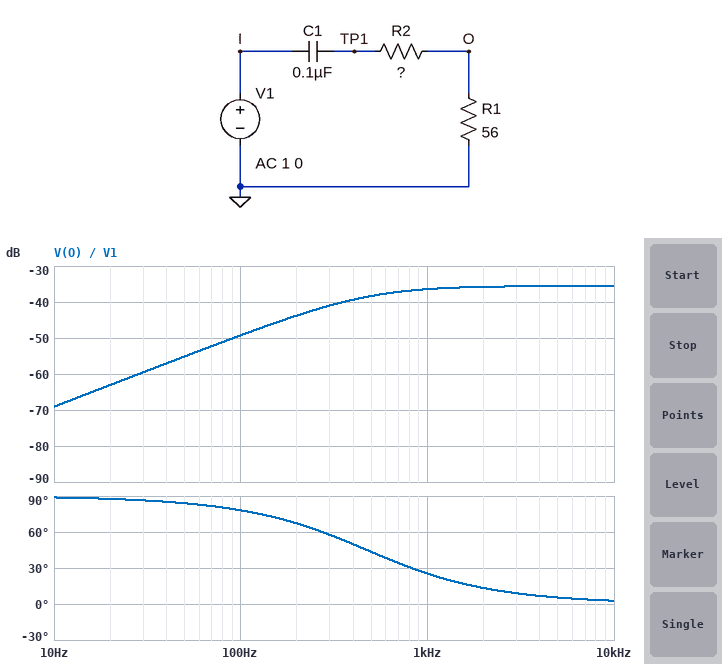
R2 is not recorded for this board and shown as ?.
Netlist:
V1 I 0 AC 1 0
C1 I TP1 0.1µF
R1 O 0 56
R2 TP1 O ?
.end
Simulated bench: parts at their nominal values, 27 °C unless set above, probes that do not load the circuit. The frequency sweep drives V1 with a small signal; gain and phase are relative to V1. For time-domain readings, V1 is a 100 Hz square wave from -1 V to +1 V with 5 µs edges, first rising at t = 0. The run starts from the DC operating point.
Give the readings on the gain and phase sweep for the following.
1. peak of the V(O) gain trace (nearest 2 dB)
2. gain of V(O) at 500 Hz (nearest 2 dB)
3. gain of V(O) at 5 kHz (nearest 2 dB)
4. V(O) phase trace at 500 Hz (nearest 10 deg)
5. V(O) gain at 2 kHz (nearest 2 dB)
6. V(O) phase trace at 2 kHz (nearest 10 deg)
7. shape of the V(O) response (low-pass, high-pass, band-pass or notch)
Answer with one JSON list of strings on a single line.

["-36 dB", "-38 dB", "-36 dB", "40 deg", "-36 dB", "10 deg", "high-pass"]
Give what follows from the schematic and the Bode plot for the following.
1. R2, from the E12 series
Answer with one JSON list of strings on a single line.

["3.3 kΩ"]
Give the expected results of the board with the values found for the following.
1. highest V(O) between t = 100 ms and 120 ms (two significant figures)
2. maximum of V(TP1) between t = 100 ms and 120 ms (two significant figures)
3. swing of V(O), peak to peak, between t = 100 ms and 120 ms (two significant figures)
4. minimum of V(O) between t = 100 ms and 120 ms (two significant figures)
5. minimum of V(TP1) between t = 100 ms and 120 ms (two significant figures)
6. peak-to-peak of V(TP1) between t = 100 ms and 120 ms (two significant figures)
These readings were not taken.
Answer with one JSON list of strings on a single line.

["33 mV", "2.0 V", "66 mV", "-33 mV", "-2.0 V", "4.0 V"]
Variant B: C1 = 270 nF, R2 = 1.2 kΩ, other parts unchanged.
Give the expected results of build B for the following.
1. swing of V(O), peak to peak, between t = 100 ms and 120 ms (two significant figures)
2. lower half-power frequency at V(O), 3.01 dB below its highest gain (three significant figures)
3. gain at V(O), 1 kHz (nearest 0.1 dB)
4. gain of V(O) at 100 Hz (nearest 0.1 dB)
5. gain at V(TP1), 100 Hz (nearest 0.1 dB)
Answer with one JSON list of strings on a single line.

["180 mV", "469 Hz", "-27.9 dB", "-40.6 dB", "-13.6 dB"]
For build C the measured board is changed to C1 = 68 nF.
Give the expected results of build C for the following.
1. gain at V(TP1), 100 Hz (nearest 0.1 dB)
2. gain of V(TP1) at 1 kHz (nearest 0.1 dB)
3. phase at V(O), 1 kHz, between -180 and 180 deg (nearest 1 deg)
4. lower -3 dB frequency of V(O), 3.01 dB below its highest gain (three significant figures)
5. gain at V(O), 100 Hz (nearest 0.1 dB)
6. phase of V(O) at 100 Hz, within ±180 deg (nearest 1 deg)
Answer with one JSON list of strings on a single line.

["-17.0 dB", "-1.7 dB", "35 deg", "697 Hz", "-52.5 dB", "82 deg"]
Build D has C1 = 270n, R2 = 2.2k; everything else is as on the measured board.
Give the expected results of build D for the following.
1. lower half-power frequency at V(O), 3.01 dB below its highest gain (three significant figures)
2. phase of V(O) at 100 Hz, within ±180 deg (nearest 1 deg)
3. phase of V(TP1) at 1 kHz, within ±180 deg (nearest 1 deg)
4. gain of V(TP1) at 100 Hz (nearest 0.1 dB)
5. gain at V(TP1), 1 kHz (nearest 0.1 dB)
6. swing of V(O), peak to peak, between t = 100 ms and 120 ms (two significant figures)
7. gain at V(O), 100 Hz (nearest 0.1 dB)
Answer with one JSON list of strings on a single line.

["261 Hz", "69 deg", "15 deg", "-8.9 dB", "-0.3 dB", "99 mV", "-41.0 dB"]
